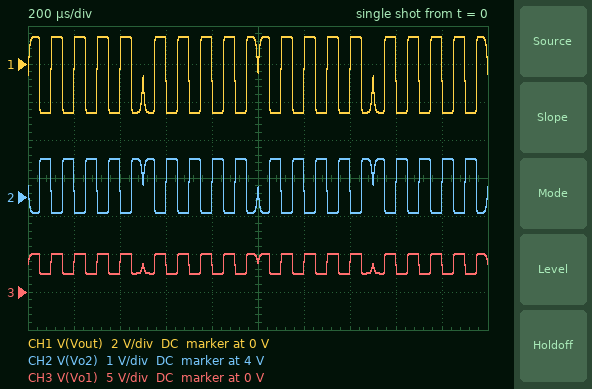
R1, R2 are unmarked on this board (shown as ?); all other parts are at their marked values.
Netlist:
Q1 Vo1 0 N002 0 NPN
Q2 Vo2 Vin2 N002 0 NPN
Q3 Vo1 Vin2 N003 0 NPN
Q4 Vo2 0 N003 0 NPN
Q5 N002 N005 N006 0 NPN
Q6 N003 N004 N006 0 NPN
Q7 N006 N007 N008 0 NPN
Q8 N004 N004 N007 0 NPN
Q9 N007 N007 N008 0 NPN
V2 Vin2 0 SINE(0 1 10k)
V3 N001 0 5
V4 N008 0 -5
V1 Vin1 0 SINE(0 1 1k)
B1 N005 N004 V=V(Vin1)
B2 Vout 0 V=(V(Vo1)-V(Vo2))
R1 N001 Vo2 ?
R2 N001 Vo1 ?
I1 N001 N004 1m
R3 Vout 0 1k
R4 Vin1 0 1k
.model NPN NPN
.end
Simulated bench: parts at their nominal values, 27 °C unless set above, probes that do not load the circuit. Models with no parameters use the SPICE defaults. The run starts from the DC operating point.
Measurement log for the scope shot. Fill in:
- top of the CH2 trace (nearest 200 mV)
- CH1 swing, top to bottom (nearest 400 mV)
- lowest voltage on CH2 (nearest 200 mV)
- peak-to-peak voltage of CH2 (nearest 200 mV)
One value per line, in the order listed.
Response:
5.0 V
4.0 V
3.6 V
1.4 V
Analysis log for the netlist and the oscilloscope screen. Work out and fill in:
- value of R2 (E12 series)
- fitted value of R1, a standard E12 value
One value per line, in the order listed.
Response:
2.7 kΩ
1.5 kΩ
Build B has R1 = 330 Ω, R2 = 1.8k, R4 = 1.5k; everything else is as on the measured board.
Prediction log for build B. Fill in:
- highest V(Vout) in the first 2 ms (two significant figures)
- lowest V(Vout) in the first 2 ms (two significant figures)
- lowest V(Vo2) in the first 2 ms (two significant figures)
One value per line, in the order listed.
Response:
310 mV
-1.7 V
4.7 V
